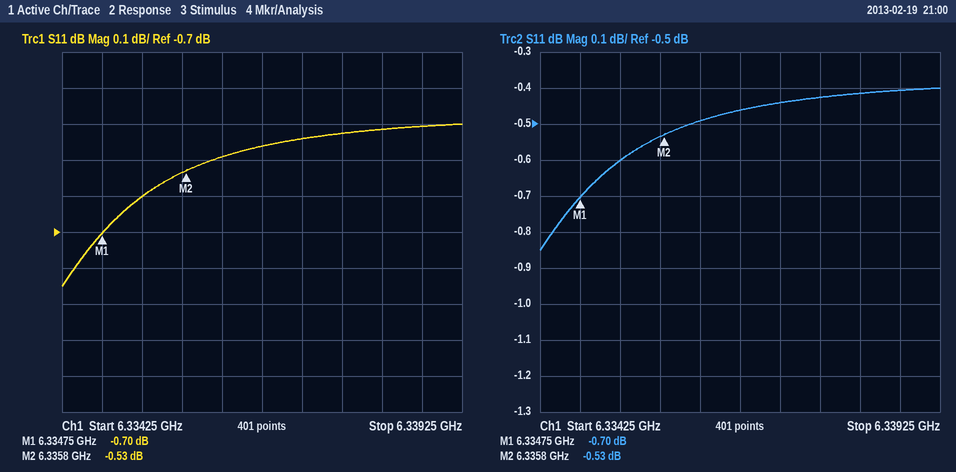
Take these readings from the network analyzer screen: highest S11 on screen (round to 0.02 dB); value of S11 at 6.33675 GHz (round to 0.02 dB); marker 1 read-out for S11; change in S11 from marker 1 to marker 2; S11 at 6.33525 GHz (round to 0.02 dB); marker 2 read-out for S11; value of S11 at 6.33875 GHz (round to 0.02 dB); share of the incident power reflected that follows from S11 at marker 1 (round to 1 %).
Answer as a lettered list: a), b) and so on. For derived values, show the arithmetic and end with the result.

a) -0.40 dB
b) -0.46 dB
c) -0.70 dB
d) -0.53 − (-0.7) = 0.17 dB
e) -0.60 dB
f) -0.53 dB
g) -0.40 dB
h) 10^(-0.7/10) ≈ 85 %
